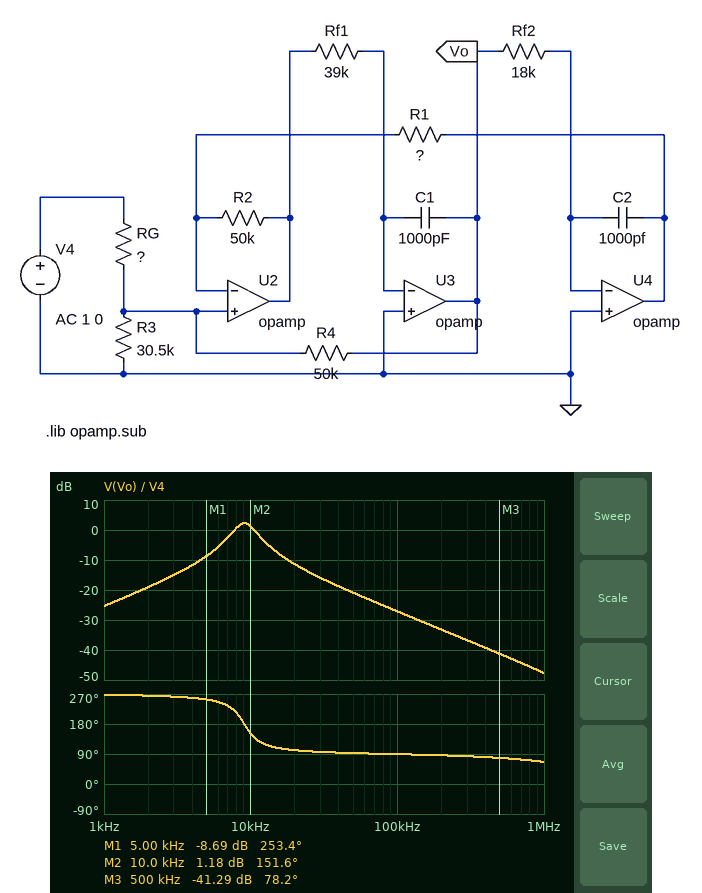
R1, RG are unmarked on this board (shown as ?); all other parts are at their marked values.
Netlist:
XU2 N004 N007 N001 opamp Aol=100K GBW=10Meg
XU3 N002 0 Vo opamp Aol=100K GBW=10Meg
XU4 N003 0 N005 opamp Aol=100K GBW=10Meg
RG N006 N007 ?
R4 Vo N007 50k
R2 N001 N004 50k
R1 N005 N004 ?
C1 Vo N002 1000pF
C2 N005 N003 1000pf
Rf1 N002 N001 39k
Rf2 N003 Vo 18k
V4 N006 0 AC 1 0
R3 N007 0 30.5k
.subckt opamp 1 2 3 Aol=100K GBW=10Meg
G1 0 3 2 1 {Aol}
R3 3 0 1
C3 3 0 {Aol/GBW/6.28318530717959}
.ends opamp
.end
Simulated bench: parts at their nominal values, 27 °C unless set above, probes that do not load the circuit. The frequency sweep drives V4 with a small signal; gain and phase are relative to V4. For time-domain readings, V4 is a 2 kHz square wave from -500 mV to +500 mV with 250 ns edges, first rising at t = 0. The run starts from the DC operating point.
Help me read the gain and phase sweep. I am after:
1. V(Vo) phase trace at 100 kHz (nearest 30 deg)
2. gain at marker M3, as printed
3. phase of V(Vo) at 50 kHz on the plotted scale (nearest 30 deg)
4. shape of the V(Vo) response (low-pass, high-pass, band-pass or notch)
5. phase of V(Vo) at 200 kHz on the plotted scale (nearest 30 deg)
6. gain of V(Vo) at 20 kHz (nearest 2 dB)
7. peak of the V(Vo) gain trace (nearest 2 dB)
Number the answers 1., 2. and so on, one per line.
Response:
1. 90 deg
2. -41.29 dB
3. 90 deg
4. band-pass
5. 90 deg
6. -12 dB
7. 2 dB
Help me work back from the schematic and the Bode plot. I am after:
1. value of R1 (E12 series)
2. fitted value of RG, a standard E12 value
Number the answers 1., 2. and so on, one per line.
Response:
1. 22 kΩ
2. 39 kΩ
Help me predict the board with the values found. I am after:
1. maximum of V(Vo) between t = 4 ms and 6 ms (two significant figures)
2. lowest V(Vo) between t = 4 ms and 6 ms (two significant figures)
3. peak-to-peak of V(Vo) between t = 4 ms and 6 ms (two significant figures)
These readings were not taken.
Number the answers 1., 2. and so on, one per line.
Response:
1. 360 mV
2. -360 mV
3. 720 mV
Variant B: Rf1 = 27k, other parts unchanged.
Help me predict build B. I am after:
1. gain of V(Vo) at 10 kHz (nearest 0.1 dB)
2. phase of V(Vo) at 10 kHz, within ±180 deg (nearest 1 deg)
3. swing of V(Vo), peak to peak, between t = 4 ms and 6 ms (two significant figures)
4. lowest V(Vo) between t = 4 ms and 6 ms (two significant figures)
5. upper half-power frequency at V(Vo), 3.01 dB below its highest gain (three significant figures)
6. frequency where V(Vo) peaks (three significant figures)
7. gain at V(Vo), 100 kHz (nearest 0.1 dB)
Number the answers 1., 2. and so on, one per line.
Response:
1. 1.7 dB
2. -159 deg
3. 870 mV
4. -430 mV
5. 13.6 kHz
6. 10.9 kHz
7. -23.9 dB
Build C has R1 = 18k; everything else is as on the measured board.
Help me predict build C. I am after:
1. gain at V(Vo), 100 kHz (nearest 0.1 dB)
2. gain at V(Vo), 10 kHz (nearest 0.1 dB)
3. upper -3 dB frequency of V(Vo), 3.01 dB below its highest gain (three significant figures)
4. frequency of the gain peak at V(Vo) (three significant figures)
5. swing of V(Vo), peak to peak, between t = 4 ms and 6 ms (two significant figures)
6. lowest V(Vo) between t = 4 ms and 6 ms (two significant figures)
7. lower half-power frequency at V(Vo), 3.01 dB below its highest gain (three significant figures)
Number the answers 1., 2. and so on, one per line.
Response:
1. -25.9 dB
2. 2.3 dB
3. 12.1 kHz
4. 10.0 kHz
5. 800 mV
6. -400 mV
7. 8.26 kHz
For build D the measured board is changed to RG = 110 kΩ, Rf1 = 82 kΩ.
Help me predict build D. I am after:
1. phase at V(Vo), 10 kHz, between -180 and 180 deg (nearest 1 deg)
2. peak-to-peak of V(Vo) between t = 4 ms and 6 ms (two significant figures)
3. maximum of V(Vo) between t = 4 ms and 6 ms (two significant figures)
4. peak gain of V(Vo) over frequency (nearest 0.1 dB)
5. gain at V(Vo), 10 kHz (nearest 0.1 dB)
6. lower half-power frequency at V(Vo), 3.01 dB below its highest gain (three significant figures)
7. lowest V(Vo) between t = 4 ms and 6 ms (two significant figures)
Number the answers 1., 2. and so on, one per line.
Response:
1. 108 deg
2. 300 mV
3. 150 mV
4. -6.8 dB
5. -16.8 dB
6. 5.31 kHz
7. -150 mV
